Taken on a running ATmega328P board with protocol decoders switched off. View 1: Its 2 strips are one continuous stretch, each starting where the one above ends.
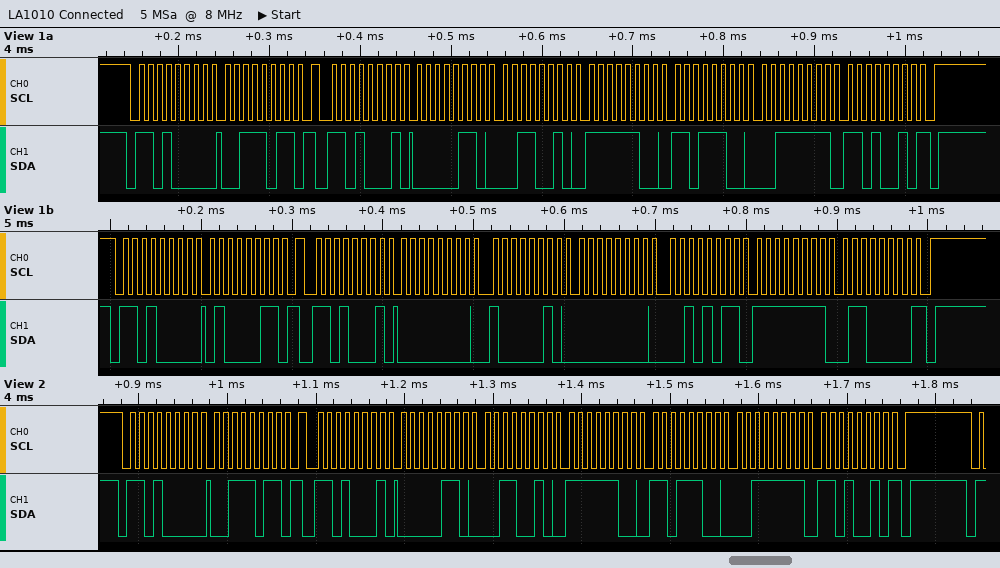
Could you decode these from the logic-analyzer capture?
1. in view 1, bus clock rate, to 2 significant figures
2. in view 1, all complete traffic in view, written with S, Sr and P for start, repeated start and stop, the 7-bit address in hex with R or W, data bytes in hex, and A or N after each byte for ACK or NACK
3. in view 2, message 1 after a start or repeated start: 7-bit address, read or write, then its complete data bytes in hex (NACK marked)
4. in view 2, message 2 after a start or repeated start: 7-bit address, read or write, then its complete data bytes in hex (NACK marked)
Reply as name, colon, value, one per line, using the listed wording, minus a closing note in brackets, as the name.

in view 1, bus clock rate, to 2 significant figures: 100 kHz
in view 1, all complete traffic in view, written with S, Sr and P for start, repeated start and stop, the 7-bit address in hex with R or W, data bytes in hex, and A or N after each byte for ACK or NACK: S 68W A 3B A Sr 68R A 06 A 32 A FC A DC A 3F A D2 N P S 68W A 43 A Sr 68R A 00 A 82 A 00 A 2B A FF A 60 N P
in view 2, message 1 after a start or repeated start: 7-bit address, read or write, then its complete data bytes in hex: 0x68 write: 3B
in view 2, message 2 after a start or repeated start: 7-bit address, read or write, then its complete data bytes in hex: 0x68 read: 06 32 FC DC 3F D2 NACK
